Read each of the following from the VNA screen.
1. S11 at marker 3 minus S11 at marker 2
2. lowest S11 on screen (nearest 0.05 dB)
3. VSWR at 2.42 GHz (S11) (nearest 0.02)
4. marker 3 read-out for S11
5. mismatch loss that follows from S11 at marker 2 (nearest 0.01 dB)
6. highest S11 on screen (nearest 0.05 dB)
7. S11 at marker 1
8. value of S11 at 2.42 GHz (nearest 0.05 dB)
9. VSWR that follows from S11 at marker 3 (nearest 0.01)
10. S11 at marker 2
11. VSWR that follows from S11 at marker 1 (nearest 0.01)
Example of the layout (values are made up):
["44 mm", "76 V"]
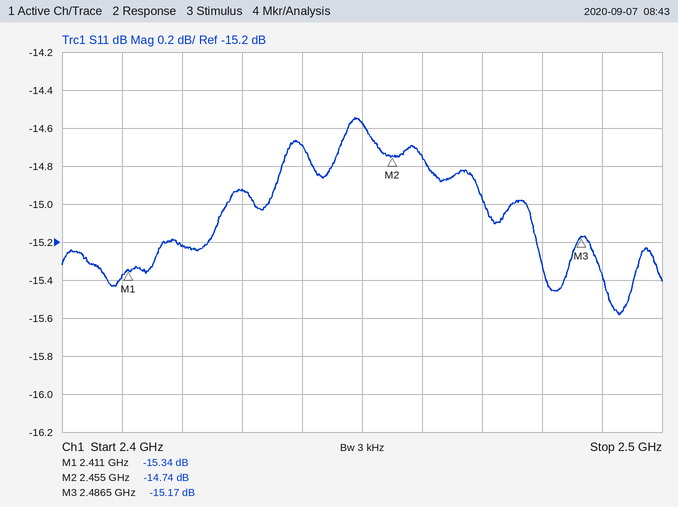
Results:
["-0.43 dB", "-15.60 dB", "1.42", "-15.17 dB", "0.15 dB", "-14.55 dB", "-15.34 dB", "-15.20 dB", "1.42", "-14.74 dB", "1.41"]
